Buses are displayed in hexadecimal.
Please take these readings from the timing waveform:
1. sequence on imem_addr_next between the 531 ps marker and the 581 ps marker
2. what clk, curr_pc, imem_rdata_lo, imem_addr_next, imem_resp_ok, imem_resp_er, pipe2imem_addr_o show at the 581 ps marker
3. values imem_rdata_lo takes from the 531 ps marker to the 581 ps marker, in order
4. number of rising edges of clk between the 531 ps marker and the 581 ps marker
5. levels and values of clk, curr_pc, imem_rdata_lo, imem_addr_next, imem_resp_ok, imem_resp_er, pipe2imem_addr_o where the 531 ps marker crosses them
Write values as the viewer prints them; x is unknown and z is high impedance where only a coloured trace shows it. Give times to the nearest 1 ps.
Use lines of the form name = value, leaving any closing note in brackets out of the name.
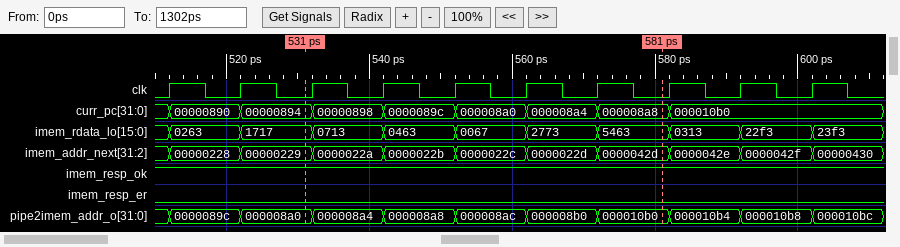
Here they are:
sequence on imem_addr_next between the 531 ps marker and the 581 ps marker = 00000229, 0000022a, 0000022b, 0000022c, 0000022d, 0000042d
what clk, curr_pc, imem_rdata_lo, imem_addr_next, imem_resp_ok, imem_resp_er, pipe2imem_addr_o show at the 581 ps marker = clk=0, curr_pc=000008a8, imem_rdata_lo=5463, imem_addr_next=0000042d, imem_resp_ok=1, imem_resp_er=0, pipe2imem_addr_o=000010b0
values imem_rdata_lo takes from the 531 ps marker to the 581 ps marker, in order = 1717, 0713, 0463, 0067, 2773, 5463
number of rising edges of clk between the 531 ps marker and the 581 ps marker = 5
levels and values of clk, curr_pc, imem_rdata_lo, imem_addr_next, imem_resp_ok, imem_resp_er, pipe2imem_addr_o where the 531 ps marker crosses them = clk=0, curr_pc=00000894, imem_rdata_lo=1717, imem_addr_next=00000229, imem_resp_ok=1, imem_resp_er=0, pipe2imem_addr_o=000008a0
